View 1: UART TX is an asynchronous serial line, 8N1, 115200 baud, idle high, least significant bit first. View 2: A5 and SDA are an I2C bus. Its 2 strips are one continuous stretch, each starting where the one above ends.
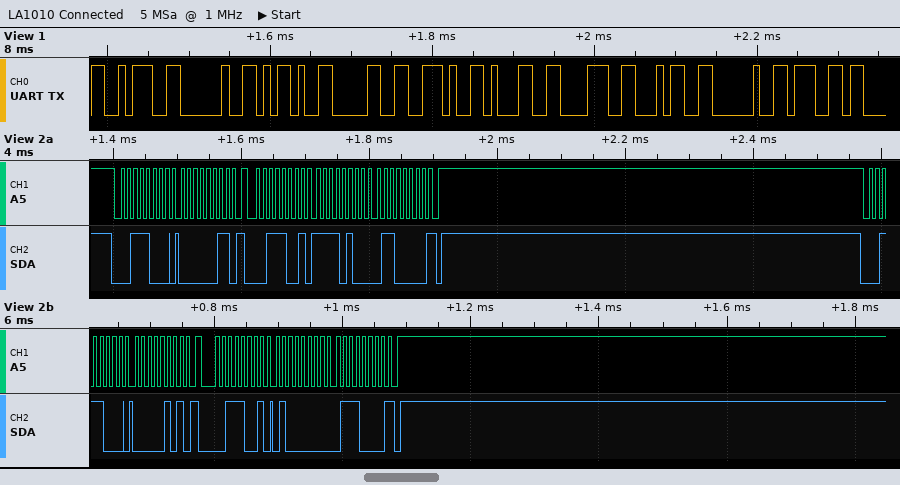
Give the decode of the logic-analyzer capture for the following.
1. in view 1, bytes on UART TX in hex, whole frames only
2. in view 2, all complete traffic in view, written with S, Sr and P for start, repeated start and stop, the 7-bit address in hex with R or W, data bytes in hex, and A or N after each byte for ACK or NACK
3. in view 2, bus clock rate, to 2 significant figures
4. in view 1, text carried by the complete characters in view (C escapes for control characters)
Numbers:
3A 20 2D 30 2E 31 38 34 20 67
S 1CW A 03 A Sr 1CR A F4 A 60 N P S 1CW A 05 A Sr 1CR A 40 A 70 N P
100 kHz
": -0.184 g"
